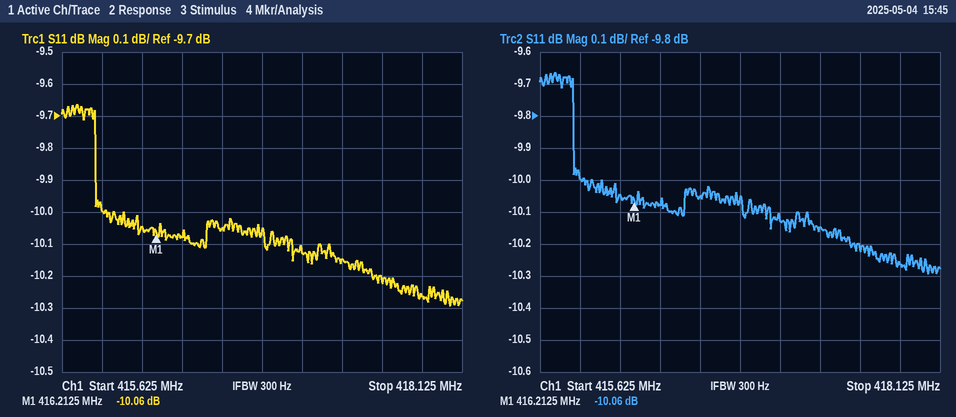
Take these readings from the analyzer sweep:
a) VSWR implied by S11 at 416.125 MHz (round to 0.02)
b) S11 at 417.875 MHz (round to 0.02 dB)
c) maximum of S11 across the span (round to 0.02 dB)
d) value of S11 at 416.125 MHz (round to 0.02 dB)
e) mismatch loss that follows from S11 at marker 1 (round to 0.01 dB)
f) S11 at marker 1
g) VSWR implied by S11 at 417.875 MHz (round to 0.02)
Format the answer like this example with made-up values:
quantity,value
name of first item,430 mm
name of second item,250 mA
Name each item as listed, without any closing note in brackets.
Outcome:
quantity,value
VSWR implied by S11 at 416.125 MHz,1.92
S11 at 417.875 MHz,-10.26 dB
maximum of S11 across the span,-9.66 dB
value of S11 at 416.125 MHz,-10.04 dB
mismatch loss that follows from S11 at marker 1,0.45 dB
S11 at marker 1,-10.06 dB
VSWR implied by S11 at 417.875 MHz,1.88
